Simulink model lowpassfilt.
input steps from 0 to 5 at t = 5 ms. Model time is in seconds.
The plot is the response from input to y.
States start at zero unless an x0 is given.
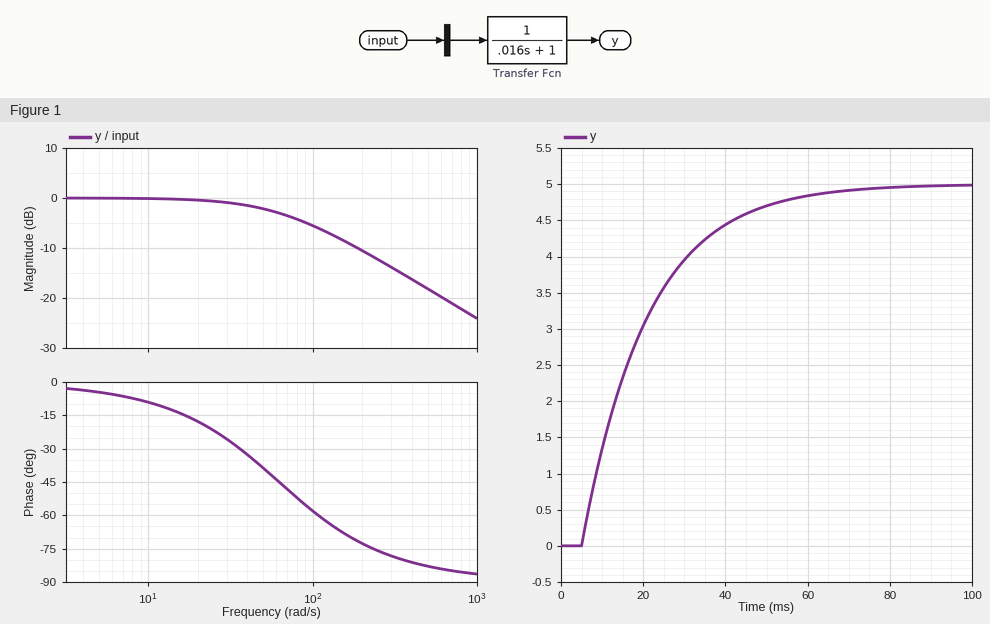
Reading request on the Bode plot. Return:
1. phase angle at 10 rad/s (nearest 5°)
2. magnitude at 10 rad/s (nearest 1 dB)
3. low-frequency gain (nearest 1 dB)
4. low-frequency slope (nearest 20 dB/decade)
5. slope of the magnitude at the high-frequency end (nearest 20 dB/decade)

-10°
0 dB
0 dB
0 dB/decade
-20 dB/decade
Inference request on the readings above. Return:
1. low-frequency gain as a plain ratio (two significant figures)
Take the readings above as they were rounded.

1.0
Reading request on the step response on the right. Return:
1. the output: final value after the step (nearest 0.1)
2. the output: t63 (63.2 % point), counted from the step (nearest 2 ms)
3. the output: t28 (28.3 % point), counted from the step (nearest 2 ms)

5.0
16 ms
6 ms
